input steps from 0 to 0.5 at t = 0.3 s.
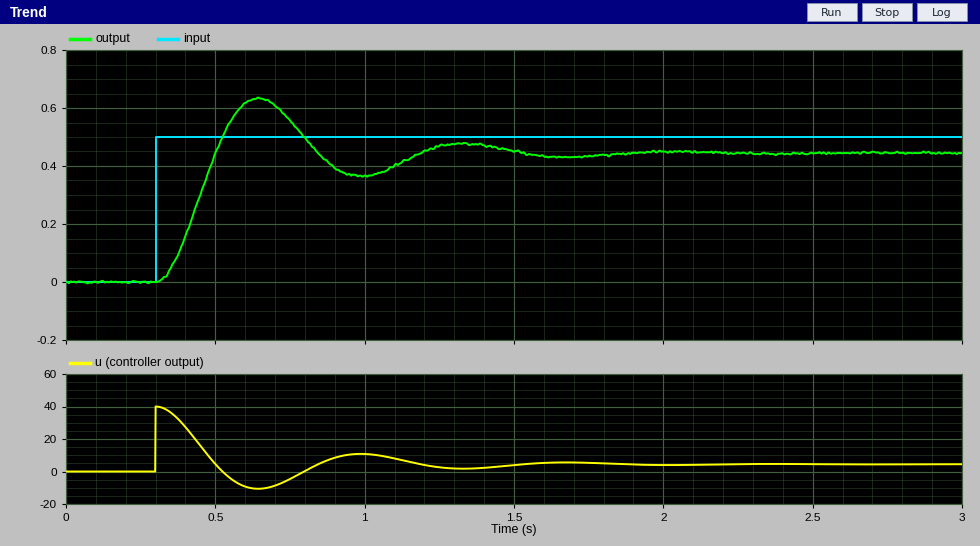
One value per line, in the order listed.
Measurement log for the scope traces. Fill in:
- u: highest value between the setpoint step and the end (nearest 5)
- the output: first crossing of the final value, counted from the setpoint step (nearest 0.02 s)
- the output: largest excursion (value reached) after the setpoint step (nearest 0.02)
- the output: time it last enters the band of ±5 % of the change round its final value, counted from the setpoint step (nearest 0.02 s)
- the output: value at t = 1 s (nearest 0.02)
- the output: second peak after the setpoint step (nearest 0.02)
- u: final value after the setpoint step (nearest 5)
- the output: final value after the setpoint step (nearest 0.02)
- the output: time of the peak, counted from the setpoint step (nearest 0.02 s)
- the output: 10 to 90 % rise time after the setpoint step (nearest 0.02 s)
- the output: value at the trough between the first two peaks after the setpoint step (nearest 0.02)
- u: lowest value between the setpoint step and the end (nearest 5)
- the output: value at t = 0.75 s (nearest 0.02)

40
0.20 s
0.64
1.12 s
0.36
0.48
5
0.44
0.34 s
0.14 s
0.36
-10
0.56
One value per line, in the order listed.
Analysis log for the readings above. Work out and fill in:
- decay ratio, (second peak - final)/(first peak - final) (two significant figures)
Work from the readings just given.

0.20
